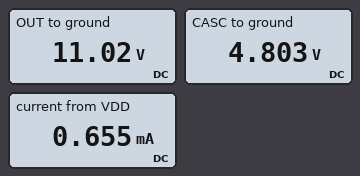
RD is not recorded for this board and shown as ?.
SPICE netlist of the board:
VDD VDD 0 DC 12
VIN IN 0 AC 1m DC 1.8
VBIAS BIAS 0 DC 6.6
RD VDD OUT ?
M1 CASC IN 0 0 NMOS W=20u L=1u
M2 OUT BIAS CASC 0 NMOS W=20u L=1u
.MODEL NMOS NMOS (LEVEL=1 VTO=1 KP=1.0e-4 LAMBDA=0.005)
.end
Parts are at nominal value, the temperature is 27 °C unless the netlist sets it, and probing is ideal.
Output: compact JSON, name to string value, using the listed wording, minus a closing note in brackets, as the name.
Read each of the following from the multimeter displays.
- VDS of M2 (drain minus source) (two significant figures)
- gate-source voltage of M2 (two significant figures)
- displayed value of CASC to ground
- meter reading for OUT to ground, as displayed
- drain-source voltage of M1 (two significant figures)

{"VDS of M2 (drain minus source)": "6.2 V", "gate-source voltage of M2": "1.8 V", "displayed value of CASC to ground": "4.803 V", "meter reading for OUT to ground, as displayed": "11.02 V", "drain-source voltage of M1": "4.8 V"}
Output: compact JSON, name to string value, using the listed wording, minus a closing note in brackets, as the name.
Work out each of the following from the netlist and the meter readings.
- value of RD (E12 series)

{"value of RD": "1.5 kΩ"}
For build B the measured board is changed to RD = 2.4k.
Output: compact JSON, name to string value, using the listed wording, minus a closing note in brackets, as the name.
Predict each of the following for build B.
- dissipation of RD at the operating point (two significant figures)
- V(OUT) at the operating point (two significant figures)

{"dissipation of RD at the operating point": "1.0 mW", "V(OUT) at the operating point": "10 V"}
